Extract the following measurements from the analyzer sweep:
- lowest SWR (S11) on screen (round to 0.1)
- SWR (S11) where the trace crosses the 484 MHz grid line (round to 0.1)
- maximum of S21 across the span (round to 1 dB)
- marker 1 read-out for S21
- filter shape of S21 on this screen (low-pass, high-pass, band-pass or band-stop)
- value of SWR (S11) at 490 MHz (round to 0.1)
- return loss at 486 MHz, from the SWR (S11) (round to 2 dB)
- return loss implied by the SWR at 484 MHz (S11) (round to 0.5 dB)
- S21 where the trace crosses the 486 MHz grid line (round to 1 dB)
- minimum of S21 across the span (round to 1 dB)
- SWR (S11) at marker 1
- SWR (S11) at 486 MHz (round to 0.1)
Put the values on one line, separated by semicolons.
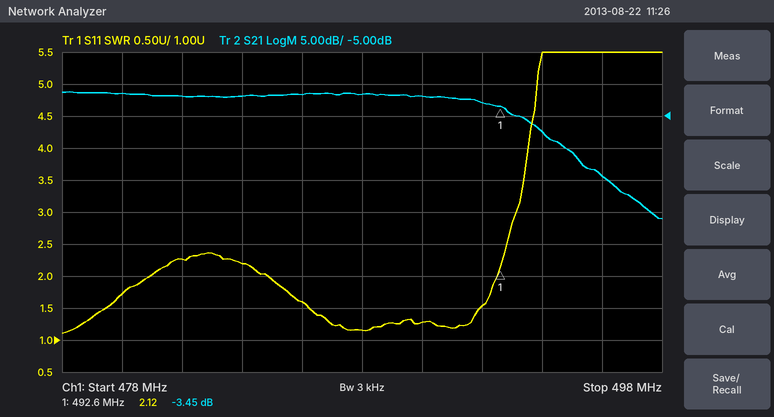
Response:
1.1; 2.2; -1 dB; -3.45 dB; low-pass; 1.3; 12 dB; 8.5 dB; -2 dB; -21 dB; 2.12; 1.6
